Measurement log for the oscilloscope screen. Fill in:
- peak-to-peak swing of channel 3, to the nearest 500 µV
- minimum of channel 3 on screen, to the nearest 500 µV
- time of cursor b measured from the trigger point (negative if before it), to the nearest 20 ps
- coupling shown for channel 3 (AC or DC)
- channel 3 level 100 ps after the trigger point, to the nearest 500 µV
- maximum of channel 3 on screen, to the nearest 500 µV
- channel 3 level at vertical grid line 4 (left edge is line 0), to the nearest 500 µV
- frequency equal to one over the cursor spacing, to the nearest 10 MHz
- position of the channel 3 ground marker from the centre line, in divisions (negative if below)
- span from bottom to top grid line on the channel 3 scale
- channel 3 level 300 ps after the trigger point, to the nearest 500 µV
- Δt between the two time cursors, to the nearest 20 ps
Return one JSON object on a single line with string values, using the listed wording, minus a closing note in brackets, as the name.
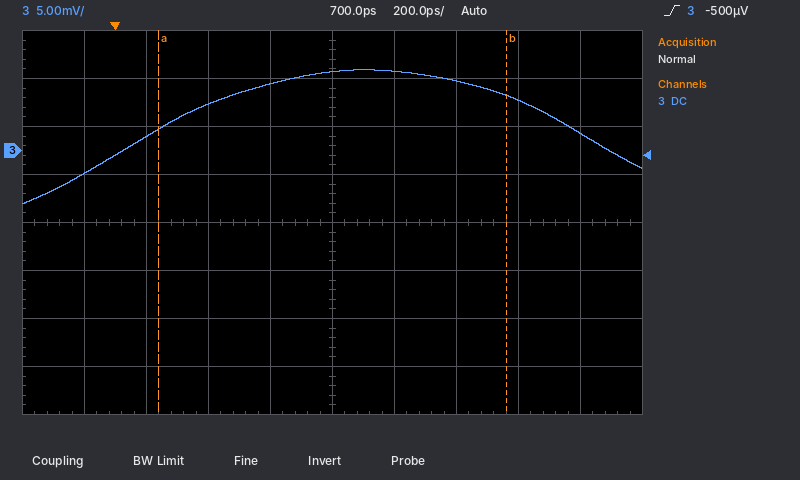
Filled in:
{"peak-to-peak swing of channel 3, to the nearest 500 µV": "14.0 mV", "minimum of channel 3 on screen, to the nearest 500 µV": "-5.5 mV", "time of cursor b measured from the trigger point (negative if before it), to the nearest 20 ps": "+1.26 ns", "coupling shown for channel 3": "DC", "channel 3 level 100 ps after the trigger point, to the nearest 500 µV": "1.5 mV", "maximum of channel 3 on screen, to the nearest 500 µV": "8.5 mV", "channel 3 level at vertical grid line 4 (left edge is line 0), to the nearest 500 µV": "7.0 mV", "frequency equal to one over the cursor spacing, to the nearest 10 MHz": "890 MHz", "position of the channel 3 ground marker from the centre line, in divisions": "+1.5 div", "span from bottom to top grid line on the channel 3 scale": "40 mV", "channel 3 level 300 ps after the trigger point, to the nearest 500 µV": "5.0 mV", "Δt between the two time cursors, to the nearest 20 ps": "1.12 ns"}
